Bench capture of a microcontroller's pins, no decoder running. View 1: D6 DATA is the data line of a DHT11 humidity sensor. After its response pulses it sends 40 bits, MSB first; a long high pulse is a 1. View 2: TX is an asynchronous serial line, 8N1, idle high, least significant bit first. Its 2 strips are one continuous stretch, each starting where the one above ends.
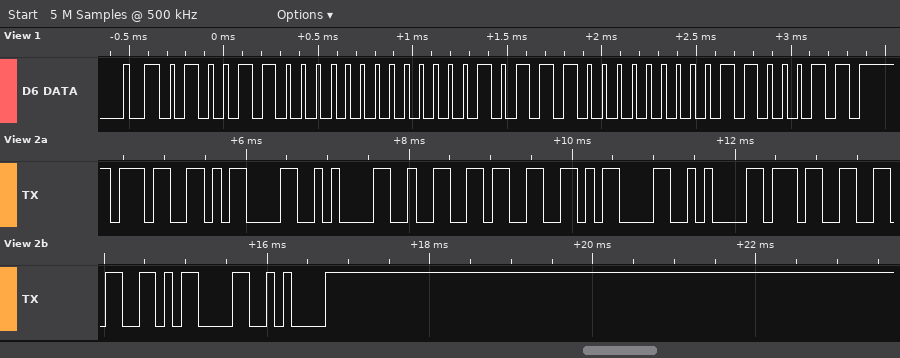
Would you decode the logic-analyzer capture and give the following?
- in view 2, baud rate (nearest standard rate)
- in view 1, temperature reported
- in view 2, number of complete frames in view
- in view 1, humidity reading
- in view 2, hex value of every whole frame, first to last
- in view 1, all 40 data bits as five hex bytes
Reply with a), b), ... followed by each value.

a) 9600 baud
b) 23.0 °C
c) 11
d) 76 %
e) 37 0D 0A 32 33 0D 0A 37 36 0D 0A
f) 4C 00 17 00 63
